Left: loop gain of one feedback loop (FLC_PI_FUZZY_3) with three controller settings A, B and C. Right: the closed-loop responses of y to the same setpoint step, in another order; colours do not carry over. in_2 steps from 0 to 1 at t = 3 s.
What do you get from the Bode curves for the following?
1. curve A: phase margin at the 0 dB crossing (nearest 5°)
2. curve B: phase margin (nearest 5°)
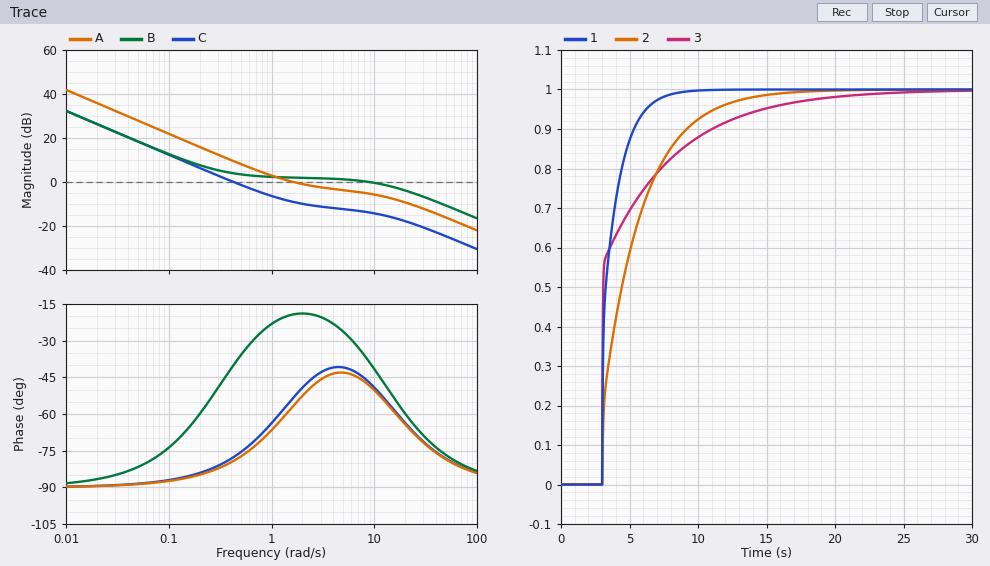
125°
140°
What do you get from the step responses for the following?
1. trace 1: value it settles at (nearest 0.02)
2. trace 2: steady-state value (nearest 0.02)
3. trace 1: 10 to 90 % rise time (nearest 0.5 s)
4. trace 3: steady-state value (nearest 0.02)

1.00
1.00
2.5 s
1.00
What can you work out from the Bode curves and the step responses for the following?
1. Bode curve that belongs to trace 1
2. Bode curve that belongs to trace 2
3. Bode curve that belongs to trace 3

A
C
B
